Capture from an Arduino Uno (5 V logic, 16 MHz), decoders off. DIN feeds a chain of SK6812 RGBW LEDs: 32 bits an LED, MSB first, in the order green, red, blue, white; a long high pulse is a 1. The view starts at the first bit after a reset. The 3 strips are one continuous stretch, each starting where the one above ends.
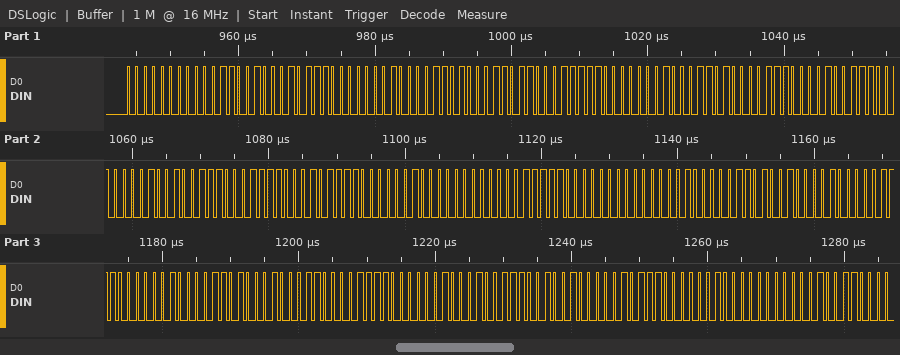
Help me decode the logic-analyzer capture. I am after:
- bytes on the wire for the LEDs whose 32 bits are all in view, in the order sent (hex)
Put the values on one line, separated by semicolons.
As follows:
00 19 17 01 0D 1B 1F 01 1A 1C 27 01 27 1E 2F 02 00 1F 00 02 0D 21 07 02 1A 23 0F 02 27 24 17 02
